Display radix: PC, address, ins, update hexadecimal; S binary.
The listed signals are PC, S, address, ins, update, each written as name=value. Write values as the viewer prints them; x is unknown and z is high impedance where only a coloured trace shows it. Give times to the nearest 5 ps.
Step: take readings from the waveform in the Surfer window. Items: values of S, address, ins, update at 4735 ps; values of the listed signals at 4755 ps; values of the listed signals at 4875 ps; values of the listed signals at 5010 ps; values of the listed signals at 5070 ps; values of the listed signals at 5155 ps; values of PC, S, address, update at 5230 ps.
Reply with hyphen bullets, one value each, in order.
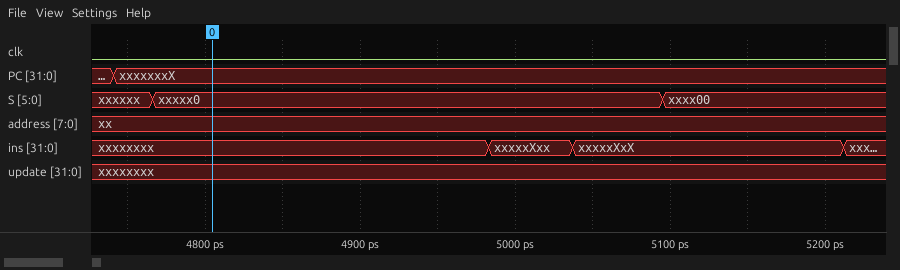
- S=xxxxxx, address=xx, ins=xxxxxxxx, update=xxxxxxxx
- PC=xxxxxxxX, S=xxxxxx, address=xx, ins=xxxxxxxx, update=xxxxxxxx
- PC=xxxxxxxX, S=xxxxx0, address=xx, ins=xxxxxxxx, update=xxxxxxxx
- PC=xxxxxxxX, S=xxxxx0, address=xx, ins=xxxxxXxx, update=xxxxxxxx
- PC=xxxxxxxX, S=xxxxx0, address=xx, ins=xxxxxXxX, update=xxxxxxxx
- PC=xxxxxxxX, S=xxxx00, address=xx, ins=xxxxxXxX, update=xxxxxxxx
- PC=xxxxxxxX, S=xxxx00, address=xx, update=xxxxxxxx
